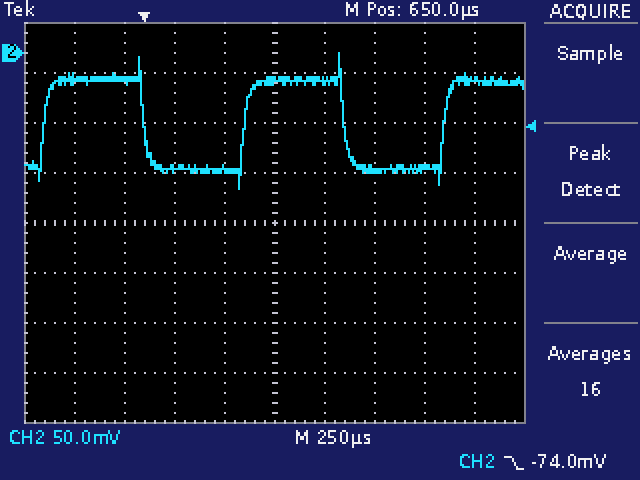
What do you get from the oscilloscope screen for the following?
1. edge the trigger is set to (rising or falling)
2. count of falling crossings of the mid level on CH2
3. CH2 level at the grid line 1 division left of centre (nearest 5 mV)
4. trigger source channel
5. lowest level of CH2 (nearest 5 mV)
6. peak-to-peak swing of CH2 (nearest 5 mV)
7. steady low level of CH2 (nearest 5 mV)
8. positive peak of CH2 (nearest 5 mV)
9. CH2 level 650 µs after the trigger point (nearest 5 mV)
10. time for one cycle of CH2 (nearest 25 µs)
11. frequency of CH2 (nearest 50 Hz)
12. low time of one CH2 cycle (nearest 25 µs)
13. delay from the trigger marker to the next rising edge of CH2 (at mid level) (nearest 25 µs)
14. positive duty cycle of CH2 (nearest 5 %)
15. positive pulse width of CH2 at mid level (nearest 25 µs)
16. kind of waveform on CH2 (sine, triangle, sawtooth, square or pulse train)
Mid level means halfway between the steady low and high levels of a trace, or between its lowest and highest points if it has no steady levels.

falling
2
-115 mV
CH2
-135 mV
135 mV
-115 mV
0 mV
-30 mV
1.000 ms
1.00 kHz
500 µs
500 µs
50 %
500 µs
square
